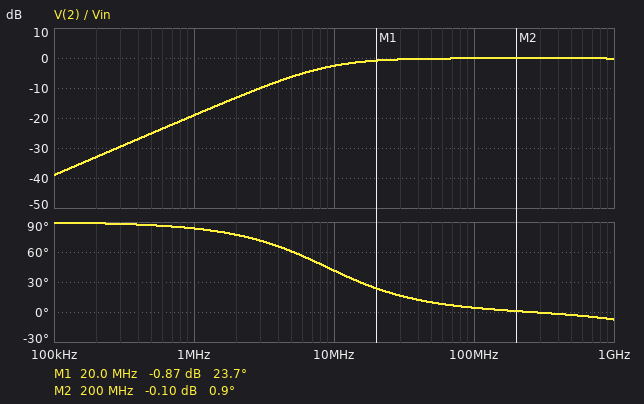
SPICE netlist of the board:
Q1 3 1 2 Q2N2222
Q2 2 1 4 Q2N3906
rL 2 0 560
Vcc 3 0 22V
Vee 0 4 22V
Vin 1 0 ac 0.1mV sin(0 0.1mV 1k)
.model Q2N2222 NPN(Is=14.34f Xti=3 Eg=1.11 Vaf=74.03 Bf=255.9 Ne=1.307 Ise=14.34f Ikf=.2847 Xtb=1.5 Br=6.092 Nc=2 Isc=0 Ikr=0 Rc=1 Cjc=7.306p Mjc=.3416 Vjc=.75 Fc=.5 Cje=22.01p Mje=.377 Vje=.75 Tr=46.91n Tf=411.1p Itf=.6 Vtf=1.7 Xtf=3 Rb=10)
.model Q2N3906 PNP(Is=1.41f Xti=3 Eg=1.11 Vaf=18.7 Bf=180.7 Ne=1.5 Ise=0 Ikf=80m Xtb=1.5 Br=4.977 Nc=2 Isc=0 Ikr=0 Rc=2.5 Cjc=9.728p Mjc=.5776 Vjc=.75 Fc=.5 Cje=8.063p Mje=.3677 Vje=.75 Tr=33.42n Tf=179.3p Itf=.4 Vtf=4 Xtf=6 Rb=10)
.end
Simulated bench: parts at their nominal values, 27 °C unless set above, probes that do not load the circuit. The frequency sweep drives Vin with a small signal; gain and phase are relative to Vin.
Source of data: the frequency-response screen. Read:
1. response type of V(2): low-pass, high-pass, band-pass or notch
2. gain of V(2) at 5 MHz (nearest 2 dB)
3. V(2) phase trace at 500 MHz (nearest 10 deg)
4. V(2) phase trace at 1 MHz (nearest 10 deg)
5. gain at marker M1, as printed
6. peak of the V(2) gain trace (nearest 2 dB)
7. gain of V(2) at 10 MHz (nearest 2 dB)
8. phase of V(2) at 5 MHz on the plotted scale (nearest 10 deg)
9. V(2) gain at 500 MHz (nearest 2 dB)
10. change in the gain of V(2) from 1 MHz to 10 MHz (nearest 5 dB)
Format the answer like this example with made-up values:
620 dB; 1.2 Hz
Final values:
high-pass; -6 dB; 0 deg; 80 deg; -0.87 dB; 0 dB; -2 dB; 60 deg; 0 dB; 15 dB
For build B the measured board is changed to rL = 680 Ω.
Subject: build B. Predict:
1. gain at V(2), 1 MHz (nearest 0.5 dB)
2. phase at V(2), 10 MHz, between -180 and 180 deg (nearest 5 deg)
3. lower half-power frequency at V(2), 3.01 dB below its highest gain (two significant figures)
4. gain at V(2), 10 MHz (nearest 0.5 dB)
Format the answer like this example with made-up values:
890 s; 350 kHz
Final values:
-17.5 dB; 35 deg; 7.3 MHz; -2.0 dB
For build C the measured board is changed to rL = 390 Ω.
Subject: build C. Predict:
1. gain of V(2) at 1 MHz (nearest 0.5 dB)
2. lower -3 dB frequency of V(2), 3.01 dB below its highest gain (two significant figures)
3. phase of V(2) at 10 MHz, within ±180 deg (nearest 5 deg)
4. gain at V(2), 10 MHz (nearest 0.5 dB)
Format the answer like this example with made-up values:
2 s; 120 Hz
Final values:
-22.0 dB; 13 MHz; 50 deg; -4.5 dB
